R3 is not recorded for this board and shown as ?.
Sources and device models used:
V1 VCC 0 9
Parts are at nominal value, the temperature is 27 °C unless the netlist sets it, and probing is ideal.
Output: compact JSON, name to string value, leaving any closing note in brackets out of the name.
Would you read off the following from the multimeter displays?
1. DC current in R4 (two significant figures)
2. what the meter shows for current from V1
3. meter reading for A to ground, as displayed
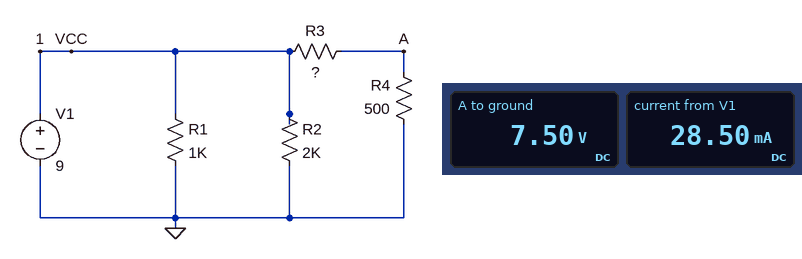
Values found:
{"DC current in R4": "15 mA", "what the meter shows for current from V1": "28.50 mA", "meter reading for A to ground, as displayed": "7.50 V"}
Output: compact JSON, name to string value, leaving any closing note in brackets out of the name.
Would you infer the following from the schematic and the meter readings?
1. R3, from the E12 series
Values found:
{"R3, from the E12 series": "100 Ω"}
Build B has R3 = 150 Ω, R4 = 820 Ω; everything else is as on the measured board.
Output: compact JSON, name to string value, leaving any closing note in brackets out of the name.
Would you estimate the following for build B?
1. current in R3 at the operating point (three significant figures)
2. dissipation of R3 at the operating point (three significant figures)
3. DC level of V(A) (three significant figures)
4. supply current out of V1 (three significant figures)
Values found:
{"current in R3 at the operating point": "9.28 mA", "dissipation of R3 at the operating point": "12.9 mW", "DC level of V(A)": "7.61 V", "supply current out of V1": "22.8 mA"}
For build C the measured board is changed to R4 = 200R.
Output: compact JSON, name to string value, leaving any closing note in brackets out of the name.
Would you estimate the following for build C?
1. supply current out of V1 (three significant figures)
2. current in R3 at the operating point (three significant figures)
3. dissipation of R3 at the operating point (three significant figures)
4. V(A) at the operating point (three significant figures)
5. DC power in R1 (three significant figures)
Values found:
{"supply current out of V1": "43.5 mA", "current in R3 at the operating point": "30.0 mA", "dissipation of R3 at the operating point": "90.0 mW", "V(A) at the operating point": "6.00 V", "DC power in R1": "81.0 mW"}
